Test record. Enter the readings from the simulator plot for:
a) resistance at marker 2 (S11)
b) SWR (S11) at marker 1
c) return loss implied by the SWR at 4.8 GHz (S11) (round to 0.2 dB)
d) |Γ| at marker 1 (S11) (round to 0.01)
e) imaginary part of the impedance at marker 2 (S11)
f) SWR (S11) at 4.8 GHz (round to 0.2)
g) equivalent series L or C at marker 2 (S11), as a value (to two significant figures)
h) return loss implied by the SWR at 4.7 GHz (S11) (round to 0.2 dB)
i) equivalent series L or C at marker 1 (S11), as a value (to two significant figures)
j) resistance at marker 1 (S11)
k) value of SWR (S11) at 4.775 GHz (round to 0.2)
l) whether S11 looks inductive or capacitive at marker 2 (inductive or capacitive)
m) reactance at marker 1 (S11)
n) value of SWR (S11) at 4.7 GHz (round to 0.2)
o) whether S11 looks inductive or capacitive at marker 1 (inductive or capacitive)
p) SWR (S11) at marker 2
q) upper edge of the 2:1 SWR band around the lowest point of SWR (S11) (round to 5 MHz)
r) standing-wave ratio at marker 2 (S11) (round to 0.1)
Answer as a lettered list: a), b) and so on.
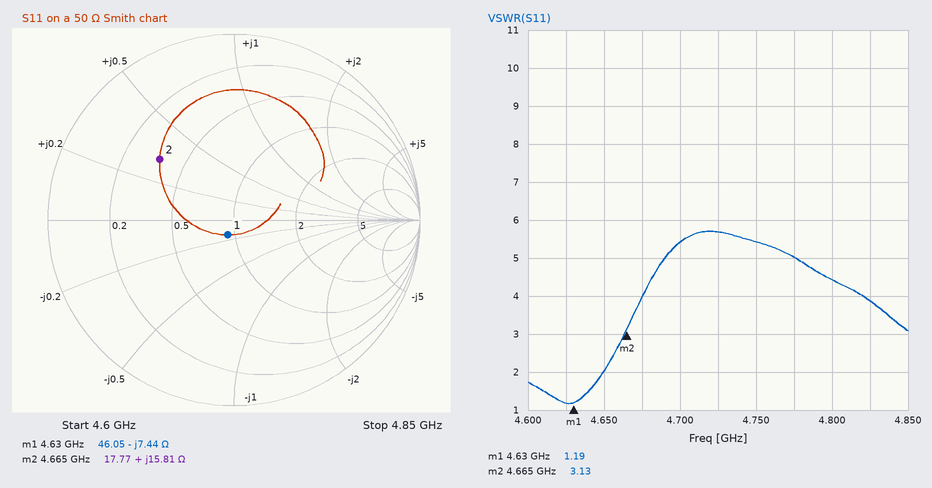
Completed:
a) 17.77 Ω
b) 1.19
c) 4.0 dB
d) 0.09
e) +15.81 Ω
f) 4.4
g) 540 pH
h) 3.2 dB
i) 4.6 pF
j) 46.05 Ω
k) 5.0
l) inductive
m) -7.44 Ω
n) 5.4
o) capacitive
p) 3.13
q) 4.650 GHz
r) 3.1
